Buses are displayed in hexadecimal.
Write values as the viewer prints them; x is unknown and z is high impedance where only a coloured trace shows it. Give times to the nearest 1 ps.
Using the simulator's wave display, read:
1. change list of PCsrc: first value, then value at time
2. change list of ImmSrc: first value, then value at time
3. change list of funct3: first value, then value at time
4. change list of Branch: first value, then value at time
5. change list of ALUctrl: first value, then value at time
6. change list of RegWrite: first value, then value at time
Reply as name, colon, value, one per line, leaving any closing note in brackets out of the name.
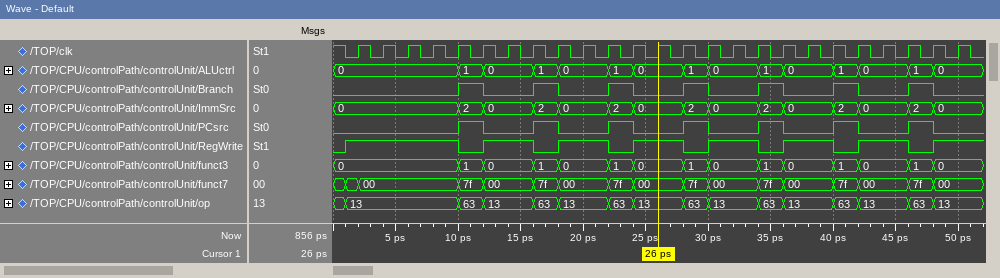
change list of PCsrc: first value, then value at time: 0, 1 at 10 ps, 0 at 12 ps, 1 at 16 ps, 0 at 18 ps, 1 at 22 ps, 0 at 24 ps, 1 at 28 ps, 0 at 30 ps, 1 at 34 ps, 0 at 36 ps, 1 at 40 ps, 0 at 42 ps, 1 at 46 ps, 0 at 48 ps
change list of ImmSrc: first value, then value at time: 0, 2 at 10 ps, 0 at 12 ps, 2 at 16 ps, 0 at 18 ps, 2 at 22 ps, 0 at 24 ps, 2 at 28 ps, 0 at 30 ps, 2 at 34 ps, 0 at 36 ps, 2 at 40 ps, 0 at 42 ps, 2 at 46 ps, 0 at 48 ps
change list of funct3: first value, then value at time: 0, 1 at 10 ps, 0 at 12 ps, 1 at 16 ps, 0 at 18 ps, 1 at 22 ps, 0 at 24 ps, 1 at 28 ps, 0 at 30 ps, 1 at 34 ps, 0 at 36 ps, 1 at 40 ps, 0 at 42 ps, 1 at 46 ps, 0 at 48 ps
change list of Branch: first value, then value at time: 0, 1 at 10 ps, 0 at 12 ps, 1 at 16 ps, 0 at 18 ps, 1 at 22 ps, 0 at 24 ps, 1 at 28 ps, 0 at 30 ps, 1 at 34 ps, 0 at 36 ps, 1 at 40 ps, 0 at 42 ps, 1 at 46 ps, 0 at 48 ps
change list of ALUctrl: first value, then value at time: 0, 1 at 10 ps, 0 at 12 ps, 1 at 16 ps, 0 at 18 ps, 1 at 22 ps, 0 at 24 ps, 1 at 28 ps, 0 at 30 ps, 1 at 34 ps, 0 at 36 ps, 1 at 40 ps, 0 at 42 ps, 1 at 46 ps, 0 at 48 ps
change list of RegWrite: first value, then value at time: 0, 1 at 1 ps, 0 at 10 ps, 1 at 12 ps, 0 at 16 ps, 1 at 18 ps, 0 at 22 ps, 1 at 24 ps, 0 at 28 ps, 1 at 30 ps, 0 at 34 ps, 1 at 36 ps, 0 at 40 ps, 1 at 42 ps, 0 at 46 ps, 1 at 48 ps
